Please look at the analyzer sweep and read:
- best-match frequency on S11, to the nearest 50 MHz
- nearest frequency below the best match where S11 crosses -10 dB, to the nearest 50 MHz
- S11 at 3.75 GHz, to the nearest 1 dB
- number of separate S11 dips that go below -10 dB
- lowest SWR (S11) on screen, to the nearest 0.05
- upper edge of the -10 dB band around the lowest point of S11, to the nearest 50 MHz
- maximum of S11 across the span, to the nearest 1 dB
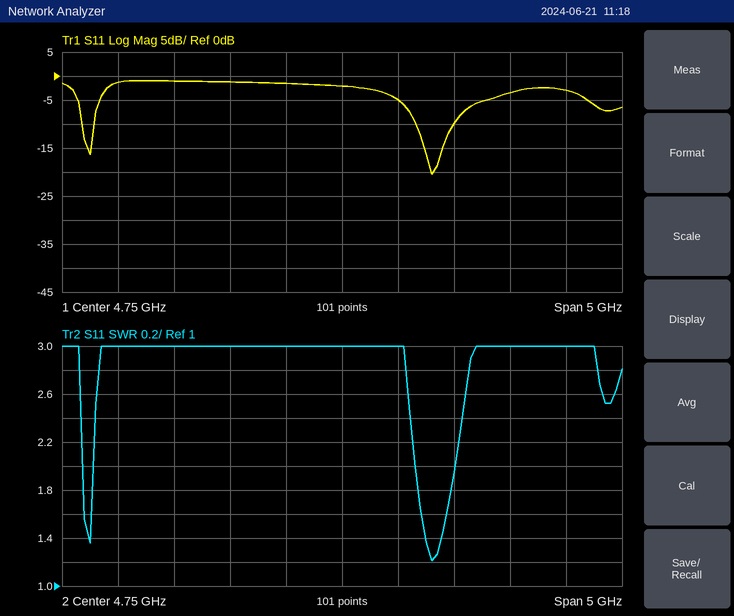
5.55 GHz
5.40 GHz
-1 dB
2
1.20
5.75 GHz
-1 dB
